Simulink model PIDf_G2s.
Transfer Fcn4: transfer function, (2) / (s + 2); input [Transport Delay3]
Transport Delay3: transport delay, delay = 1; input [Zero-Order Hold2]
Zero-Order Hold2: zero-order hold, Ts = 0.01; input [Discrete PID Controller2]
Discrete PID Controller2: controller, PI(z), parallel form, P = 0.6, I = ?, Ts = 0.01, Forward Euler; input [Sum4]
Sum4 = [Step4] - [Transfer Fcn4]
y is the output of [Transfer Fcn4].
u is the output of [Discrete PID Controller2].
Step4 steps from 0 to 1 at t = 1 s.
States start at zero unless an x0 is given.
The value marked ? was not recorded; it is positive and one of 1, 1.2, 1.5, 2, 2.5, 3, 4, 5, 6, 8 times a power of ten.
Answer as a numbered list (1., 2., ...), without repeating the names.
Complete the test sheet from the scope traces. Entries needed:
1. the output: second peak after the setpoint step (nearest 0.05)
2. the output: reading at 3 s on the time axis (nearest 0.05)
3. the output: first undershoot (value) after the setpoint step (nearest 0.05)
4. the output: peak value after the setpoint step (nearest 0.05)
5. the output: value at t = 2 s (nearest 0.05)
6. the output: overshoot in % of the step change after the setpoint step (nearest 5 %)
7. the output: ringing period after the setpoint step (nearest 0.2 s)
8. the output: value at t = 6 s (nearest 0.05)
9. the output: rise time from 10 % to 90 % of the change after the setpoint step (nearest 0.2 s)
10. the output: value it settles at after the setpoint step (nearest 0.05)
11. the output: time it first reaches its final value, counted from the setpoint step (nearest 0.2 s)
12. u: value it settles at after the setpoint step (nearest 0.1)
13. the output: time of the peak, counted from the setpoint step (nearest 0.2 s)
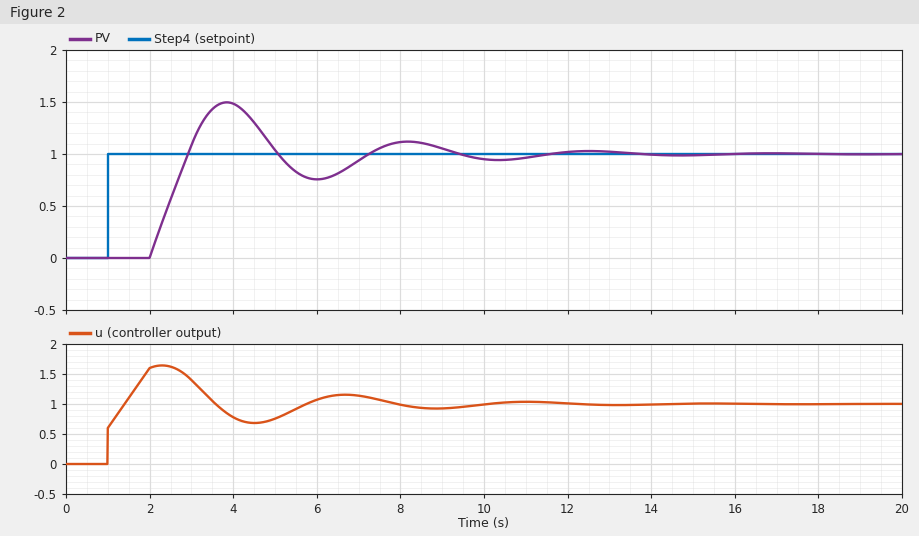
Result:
1. 1.10
2. 1.10
3. 0.75
4. 1.50
5. 0.00
6. 50 %
7. 4.4 s
8. 0.75
9. 0.8 s
10. 1.00
11. 2.0 s
12. 1.0
13. 2.8 s
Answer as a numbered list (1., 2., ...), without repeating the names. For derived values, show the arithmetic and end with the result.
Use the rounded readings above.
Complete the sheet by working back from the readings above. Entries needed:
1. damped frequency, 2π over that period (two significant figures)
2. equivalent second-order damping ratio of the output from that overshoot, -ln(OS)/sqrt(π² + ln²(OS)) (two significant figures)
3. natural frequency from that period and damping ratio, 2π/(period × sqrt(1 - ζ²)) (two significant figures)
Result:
1. 2π / 4.4 = 1.4 rad/s
2. ln(0.5) = -0.693; 0.693 / sqrt(9.870 + 0.480) = 0.22
3. 2π / (4.4 × sqrt(1 - 0.22²)) = 1.5 rad/s
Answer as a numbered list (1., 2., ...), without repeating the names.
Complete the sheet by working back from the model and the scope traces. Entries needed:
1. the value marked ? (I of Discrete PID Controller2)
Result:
1. 1
